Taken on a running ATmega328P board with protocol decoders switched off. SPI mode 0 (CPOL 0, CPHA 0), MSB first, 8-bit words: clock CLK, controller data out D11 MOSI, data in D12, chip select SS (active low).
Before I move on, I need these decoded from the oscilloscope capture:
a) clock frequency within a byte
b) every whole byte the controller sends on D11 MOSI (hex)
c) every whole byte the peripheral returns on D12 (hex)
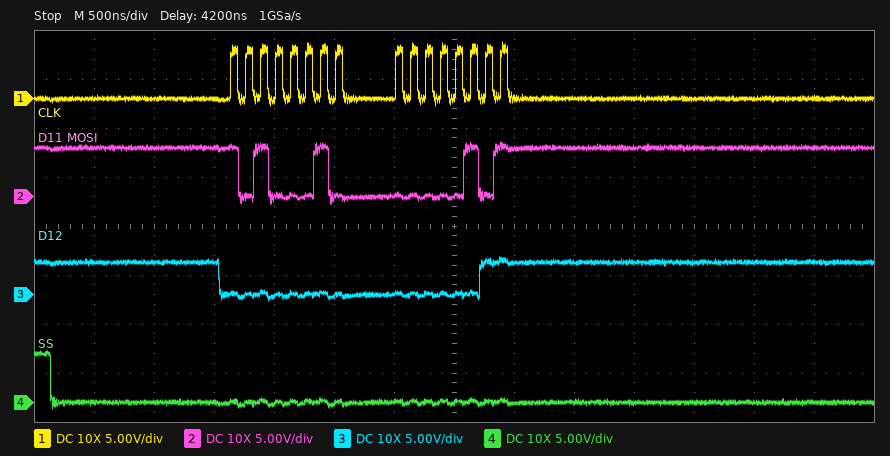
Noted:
8 MHz
0xA2 0x05
0x00 0x03
